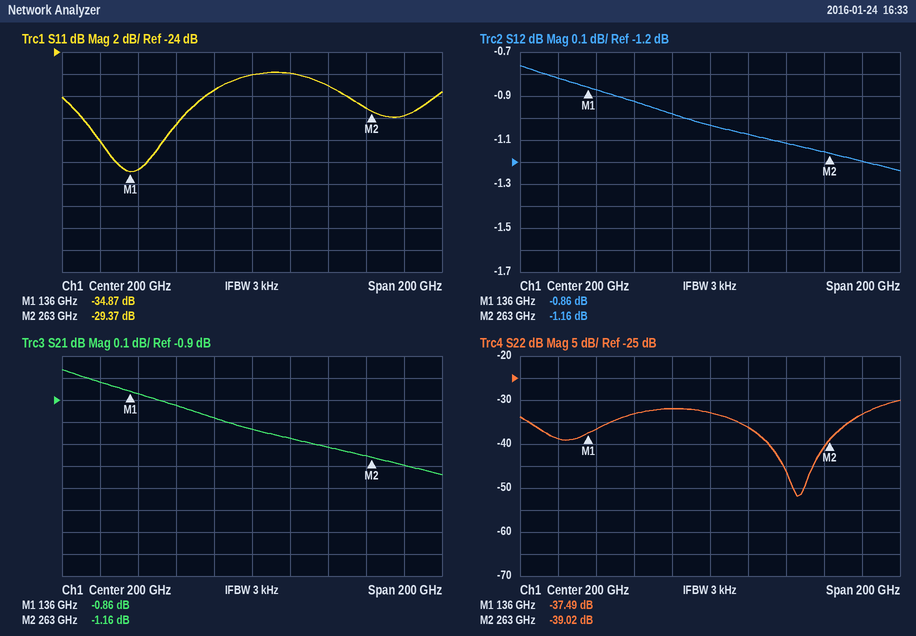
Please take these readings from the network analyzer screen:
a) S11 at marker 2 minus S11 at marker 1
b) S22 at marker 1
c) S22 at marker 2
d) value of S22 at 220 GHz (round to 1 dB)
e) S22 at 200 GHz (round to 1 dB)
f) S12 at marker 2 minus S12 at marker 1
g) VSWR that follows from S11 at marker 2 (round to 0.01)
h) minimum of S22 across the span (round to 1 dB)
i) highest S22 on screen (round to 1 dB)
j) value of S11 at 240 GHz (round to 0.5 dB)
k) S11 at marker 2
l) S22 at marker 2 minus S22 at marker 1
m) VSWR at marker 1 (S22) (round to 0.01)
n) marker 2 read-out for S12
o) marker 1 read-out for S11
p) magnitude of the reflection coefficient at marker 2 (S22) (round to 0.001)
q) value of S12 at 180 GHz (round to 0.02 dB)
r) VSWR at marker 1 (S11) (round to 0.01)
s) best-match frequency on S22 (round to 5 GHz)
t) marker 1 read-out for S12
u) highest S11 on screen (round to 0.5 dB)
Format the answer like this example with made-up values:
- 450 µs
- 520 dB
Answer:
- 5.50 dB
- -37.49 dB
- -39.02 dB
- -36 dB
- -33 dB
- -0.30 dB
- 1.07
- -52 dB
- -30 dB
- -27.0 dB
- -29.37 dB
- -1.53 dB
- 1.03
- -1.16 dB
- -34.87 dB
- 0.011
- -0.98 dB
- 1.04
- 245 GHz
- -0.86 dB
- -26.0 dB
